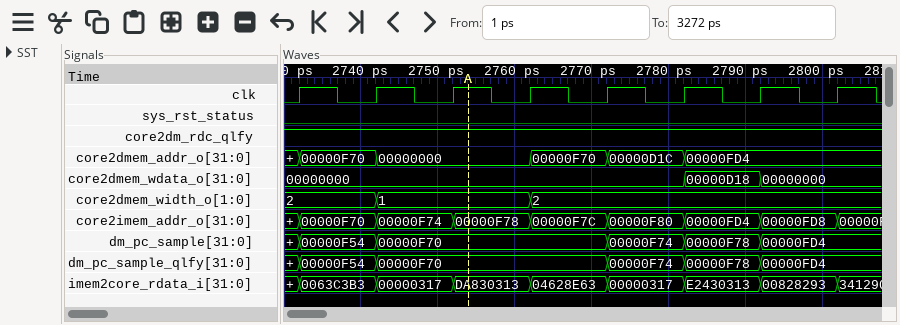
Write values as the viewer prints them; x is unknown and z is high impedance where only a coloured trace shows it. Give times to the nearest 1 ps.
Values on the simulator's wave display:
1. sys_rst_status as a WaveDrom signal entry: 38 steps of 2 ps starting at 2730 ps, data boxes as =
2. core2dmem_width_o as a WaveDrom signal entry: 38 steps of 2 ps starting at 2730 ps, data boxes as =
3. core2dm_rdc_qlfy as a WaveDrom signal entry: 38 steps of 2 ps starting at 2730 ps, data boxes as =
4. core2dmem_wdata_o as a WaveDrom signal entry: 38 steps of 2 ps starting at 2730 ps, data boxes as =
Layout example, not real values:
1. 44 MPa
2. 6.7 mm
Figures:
1. {name: 'sys_rst_status', wave: '0.....................................'}
2. {name: 'core2dmem_width_o', wave: '=.....=.........=.....................', data: '2 1 2'}
3. {name: 'core2dm_rdc_qlfy', wave: '1.....................................'}
4. {name: 'core2dmem_wdata_o', wave: '=.........................=....=......', data: '00000000 00000D18 00000000'}
